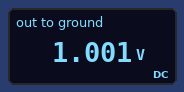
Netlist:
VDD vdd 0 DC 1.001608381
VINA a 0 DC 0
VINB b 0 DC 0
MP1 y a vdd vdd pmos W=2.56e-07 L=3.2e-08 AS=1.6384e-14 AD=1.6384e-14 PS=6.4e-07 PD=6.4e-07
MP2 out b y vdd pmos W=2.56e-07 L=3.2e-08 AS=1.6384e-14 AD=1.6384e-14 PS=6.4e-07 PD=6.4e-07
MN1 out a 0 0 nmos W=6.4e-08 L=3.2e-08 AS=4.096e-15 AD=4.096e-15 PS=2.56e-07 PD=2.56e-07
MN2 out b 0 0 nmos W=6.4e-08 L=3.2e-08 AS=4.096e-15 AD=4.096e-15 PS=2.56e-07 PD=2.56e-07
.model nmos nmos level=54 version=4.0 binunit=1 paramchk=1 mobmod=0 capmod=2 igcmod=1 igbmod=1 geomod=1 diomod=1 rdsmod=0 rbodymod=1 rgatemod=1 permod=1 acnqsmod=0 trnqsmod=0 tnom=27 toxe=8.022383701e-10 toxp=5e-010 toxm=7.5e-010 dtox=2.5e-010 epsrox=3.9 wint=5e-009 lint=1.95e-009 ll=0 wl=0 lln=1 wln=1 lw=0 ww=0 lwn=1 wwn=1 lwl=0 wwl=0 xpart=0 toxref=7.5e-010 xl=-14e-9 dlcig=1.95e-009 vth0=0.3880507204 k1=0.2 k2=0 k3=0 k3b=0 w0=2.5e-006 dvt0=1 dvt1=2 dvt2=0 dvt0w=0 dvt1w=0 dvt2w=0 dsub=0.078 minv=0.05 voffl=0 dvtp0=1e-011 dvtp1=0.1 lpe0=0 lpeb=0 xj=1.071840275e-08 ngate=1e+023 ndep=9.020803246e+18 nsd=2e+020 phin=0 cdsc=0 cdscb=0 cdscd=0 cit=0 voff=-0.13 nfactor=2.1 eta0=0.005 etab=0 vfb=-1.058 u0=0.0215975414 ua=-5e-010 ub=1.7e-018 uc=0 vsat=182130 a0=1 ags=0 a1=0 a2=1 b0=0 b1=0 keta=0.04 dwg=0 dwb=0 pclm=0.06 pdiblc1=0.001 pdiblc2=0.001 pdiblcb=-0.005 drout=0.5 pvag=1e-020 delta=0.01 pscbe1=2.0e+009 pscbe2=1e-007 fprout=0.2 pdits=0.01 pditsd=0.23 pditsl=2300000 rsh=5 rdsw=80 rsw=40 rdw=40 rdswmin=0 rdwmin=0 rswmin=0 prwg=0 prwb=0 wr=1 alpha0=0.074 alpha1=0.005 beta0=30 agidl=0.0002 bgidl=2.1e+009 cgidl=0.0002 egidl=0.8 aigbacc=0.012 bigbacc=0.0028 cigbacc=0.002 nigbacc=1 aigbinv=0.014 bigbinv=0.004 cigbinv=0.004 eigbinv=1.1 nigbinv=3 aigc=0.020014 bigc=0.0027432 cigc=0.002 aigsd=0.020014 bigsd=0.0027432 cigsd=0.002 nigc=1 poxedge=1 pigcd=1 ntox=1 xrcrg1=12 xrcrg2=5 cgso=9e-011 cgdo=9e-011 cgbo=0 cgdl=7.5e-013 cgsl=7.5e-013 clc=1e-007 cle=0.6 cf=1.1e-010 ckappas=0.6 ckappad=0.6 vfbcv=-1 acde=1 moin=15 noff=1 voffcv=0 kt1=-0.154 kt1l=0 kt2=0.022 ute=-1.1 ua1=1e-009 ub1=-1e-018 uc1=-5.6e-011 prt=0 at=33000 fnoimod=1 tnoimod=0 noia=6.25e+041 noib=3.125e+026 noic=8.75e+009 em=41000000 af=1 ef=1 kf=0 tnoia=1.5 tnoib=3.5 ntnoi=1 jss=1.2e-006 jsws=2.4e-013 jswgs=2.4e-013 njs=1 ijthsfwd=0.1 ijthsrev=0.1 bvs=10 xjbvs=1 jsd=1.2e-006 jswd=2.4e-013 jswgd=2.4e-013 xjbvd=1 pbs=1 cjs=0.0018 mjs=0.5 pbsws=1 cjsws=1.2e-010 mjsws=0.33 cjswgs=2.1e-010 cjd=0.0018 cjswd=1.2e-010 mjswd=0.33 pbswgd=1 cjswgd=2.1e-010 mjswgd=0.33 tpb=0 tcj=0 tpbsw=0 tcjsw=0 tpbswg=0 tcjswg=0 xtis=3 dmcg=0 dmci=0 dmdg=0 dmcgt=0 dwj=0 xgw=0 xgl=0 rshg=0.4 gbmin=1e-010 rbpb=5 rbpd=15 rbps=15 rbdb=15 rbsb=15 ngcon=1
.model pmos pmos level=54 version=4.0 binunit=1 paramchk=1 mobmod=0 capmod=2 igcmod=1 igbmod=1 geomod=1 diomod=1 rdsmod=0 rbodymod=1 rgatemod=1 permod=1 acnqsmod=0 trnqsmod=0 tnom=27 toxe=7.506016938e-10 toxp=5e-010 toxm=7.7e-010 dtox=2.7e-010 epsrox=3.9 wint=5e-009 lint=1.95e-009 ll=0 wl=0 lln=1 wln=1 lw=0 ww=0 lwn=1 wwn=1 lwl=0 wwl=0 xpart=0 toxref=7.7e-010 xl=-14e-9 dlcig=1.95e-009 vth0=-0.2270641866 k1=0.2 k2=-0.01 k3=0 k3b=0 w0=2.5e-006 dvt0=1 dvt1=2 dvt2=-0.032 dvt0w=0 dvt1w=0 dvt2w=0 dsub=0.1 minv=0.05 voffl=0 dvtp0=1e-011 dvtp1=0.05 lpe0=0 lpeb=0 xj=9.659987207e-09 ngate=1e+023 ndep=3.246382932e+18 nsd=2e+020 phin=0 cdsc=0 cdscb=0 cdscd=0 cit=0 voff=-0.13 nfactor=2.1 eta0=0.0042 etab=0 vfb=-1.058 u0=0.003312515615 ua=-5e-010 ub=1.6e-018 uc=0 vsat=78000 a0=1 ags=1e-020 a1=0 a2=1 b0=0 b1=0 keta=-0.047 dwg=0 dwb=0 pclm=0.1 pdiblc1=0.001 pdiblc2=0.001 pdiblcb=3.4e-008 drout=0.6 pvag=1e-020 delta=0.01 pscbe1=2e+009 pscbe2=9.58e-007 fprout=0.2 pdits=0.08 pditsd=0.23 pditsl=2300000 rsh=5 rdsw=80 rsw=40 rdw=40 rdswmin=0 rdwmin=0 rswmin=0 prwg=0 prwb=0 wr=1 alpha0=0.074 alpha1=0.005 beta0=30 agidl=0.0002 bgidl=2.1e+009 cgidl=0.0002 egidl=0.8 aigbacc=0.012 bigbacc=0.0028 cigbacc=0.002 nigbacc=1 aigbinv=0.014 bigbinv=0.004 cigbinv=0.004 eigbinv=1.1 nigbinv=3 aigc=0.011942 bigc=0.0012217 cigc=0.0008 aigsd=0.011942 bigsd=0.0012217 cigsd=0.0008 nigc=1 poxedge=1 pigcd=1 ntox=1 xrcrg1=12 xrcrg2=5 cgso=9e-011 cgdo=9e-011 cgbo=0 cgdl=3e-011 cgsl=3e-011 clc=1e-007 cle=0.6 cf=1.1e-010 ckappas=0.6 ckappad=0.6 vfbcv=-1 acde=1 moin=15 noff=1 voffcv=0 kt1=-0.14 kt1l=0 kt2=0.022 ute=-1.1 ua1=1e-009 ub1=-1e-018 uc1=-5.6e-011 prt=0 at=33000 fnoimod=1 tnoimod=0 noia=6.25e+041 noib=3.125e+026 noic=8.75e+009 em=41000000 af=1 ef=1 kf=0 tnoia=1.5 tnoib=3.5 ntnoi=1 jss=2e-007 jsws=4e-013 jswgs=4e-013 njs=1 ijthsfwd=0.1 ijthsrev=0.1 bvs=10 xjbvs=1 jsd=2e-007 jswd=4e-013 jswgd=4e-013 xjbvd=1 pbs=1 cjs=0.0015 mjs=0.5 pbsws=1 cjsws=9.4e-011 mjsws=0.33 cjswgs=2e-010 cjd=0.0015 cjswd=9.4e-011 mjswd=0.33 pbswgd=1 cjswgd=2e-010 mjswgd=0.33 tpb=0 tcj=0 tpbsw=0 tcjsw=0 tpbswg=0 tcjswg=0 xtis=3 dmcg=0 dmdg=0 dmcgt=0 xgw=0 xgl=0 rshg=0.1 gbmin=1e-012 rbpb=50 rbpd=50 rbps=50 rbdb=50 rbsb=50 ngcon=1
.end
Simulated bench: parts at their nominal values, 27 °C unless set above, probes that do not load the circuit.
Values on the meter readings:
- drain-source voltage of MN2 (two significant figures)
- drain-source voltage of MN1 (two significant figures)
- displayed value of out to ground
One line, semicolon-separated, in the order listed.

1.0 V; 1.0 V; 1.001 V
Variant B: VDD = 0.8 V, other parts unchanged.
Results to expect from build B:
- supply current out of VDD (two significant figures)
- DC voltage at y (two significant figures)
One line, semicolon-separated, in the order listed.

170 nA; 800 mV
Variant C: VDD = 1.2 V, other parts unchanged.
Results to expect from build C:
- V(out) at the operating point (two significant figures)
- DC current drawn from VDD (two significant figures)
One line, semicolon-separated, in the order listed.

1.2 V; 1.2 µA
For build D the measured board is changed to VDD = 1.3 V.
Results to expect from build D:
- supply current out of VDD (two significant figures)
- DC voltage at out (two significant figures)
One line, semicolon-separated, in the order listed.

2.5 µA; 1.3 V
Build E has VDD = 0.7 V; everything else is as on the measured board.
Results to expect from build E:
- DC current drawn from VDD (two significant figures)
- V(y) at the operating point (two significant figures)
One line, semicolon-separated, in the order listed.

110 nA; 700 mV
